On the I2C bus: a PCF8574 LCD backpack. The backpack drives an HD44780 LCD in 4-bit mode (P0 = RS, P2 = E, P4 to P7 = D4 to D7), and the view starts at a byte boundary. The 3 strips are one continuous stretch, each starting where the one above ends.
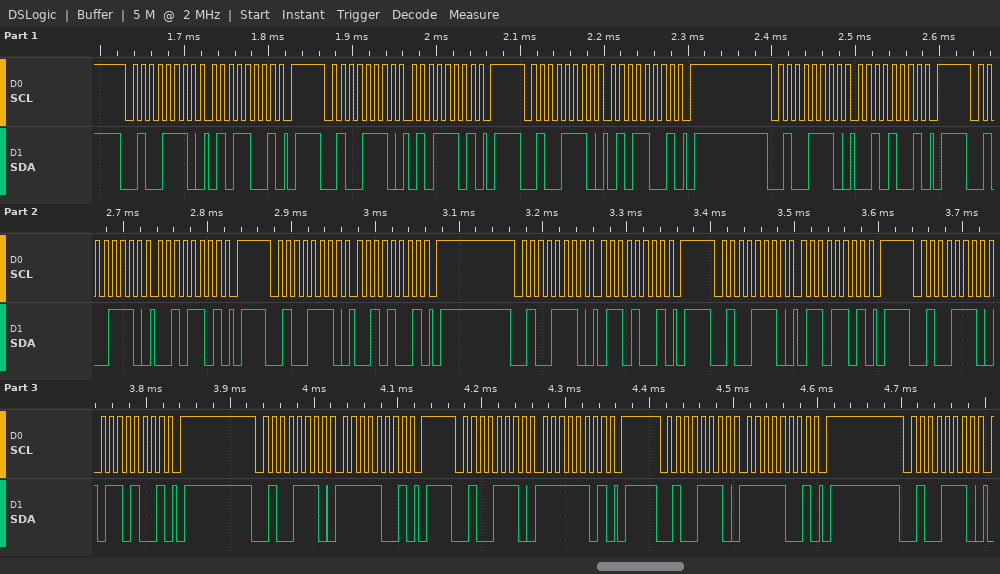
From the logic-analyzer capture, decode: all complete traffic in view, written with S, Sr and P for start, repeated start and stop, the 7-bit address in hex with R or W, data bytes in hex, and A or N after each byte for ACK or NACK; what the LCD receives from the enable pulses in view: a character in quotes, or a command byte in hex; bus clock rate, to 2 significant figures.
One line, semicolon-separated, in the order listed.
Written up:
S 27W A 59 A P S 27W A 5D A P S 27W A 59 A P S 27W A 29 A P S 27W A 2D A P S 27W A 29 A P S 27W A 69 A P S 27W A 6D A P S 27W A 69 A P S 27W A F9 A P S 27W A FD A P S 27W A F9 A P S 27W A; 'R' 'o'; 100 kHz
